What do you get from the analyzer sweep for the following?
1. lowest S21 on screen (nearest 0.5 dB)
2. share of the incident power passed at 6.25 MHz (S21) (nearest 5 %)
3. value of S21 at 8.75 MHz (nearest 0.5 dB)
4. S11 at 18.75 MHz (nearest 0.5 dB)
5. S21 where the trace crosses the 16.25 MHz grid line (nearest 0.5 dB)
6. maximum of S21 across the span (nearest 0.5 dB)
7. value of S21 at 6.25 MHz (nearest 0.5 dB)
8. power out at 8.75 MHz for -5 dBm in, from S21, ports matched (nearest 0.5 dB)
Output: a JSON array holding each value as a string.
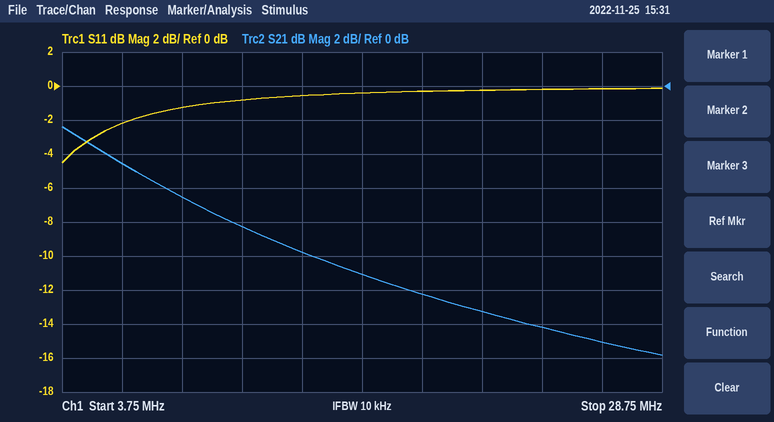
["-16.0 dB", "35 %", "-6.5 dB", "-0.5 dB", "-11.0 dB", "-2.5 dB", "-4.5 dB", "-11.5 dBm"]
